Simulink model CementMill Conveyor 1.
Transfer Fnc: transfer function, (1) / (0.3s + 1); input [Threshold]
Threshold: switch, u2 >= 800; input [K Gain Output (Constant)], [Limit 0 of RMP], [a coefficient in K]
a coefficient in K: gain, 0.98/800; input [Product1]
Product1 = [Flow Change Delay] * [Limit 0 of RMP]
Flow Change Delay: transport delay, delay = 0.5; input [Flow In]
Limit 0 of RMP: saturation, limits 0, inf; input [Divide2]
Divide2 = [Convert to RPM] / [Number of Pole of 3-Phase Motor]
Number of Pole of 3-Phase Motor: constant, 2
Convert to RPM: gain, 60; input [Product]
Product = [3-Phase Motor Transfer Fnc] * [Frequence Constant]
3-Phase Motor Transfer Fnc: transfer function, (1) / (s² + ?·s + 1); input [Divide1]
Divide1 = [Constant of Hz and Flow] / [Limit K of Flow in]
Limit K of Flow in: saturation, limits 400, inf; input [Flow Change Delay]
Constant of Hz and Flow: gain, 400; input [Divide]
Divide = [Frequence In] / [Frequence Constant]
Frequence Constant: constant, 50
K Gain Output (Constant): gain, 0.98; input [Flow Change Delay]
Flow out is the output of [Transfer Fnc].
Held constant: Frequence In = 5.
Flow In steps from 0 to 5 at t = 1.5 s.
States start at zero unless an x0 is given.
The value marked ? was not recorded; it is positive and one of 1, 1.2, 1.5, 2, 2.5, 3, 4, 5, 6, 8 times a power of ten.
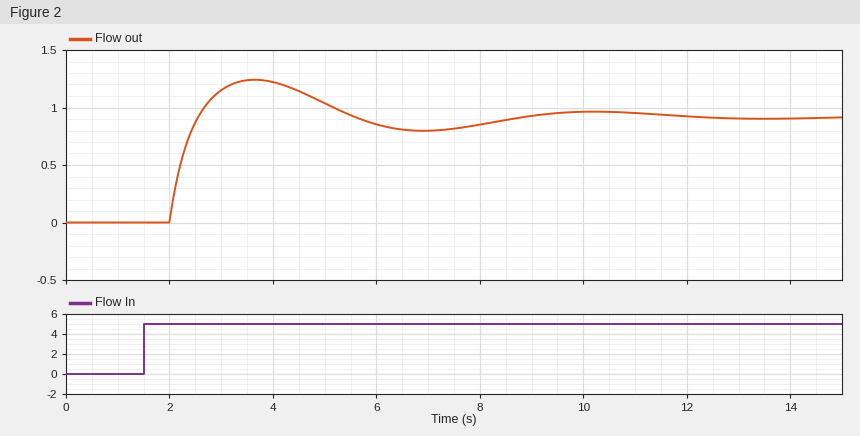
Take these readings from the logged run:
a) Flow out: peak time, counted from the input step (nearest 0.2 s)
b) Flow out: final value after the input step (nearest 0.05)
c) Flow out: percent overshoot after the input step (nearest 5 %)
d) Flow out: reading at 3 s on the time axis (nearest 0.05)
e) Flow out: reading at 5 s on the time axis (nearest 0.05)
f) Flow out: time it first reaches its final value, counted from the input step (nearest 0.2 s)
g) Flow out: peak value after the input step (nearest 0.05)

2.2 s
0.90
35 %
1.15
1.05
1.0 s
1.25
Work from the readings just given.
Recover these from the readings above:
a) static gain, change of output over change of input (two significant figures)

0.18
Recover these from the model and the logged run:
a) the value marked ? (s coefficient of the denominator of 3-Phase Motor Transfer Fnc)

0.6
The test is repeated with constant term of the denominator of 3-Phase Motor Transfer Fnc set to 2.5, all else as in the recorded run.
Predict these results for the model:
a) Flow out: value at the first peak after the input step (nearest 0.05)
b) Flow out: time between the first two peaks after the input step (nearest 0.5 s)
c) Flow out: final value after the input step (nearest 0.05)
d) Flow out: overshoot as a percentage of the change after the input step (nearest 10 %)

0.45
3.5 s
0.35
30 %
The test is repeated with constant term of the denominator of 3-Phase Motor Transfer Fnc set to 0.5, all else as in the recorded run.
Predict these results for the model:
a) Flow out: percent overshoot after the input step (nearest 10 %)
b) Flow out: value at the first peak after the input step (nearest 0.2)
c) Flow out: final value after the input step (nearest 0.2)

20 %
2.2
1.8
